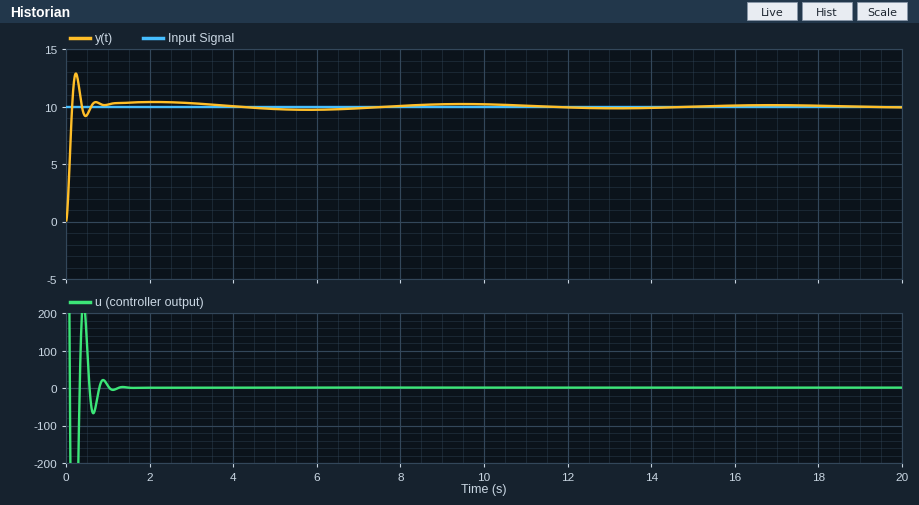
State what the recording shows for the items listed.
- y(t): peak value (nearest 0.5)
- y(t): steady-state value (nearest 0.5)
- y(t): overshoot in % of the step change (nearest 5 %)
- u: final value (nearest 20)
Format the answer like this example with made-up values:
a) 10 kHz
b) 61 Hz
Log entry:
a) 13.0
b) 10.0
c) 30 %
d) 0
